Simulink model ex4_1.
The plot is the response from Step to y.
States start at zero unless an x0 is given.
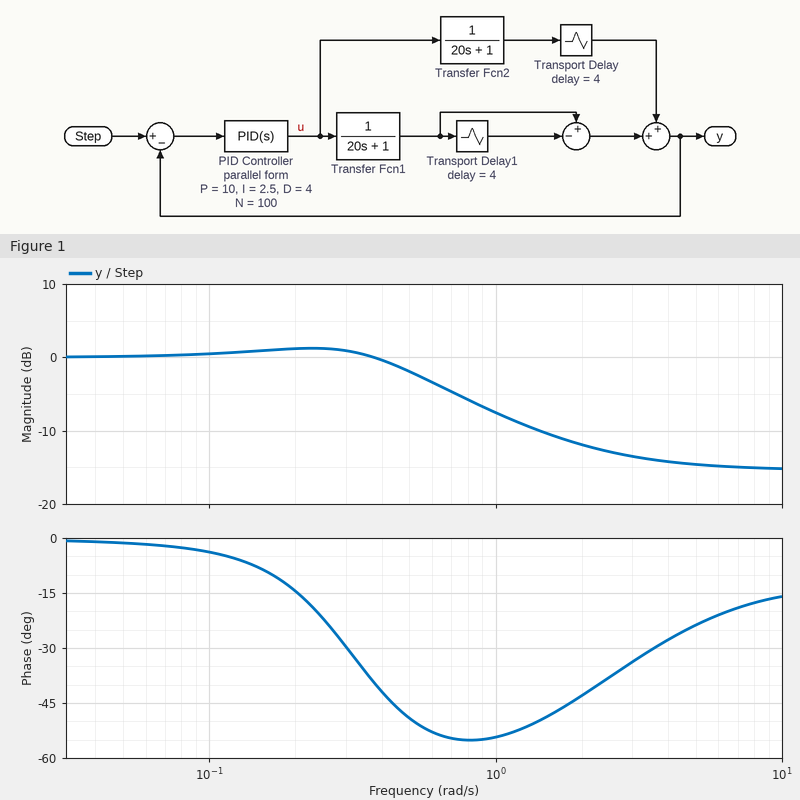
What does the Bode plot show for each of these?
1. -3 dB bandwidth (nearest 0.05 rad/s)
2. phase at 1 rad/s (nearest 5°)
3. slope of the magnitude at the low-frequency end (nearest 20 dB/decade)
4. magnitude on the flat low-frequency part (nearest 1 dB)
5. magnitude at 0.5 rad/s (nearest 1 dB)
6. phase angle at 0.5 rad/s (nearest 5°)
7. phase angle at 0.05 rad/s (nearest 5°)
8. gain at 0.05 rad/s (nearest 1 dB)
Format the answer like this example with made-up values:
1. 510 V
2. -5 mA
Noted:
1. 0.55 rad/s
2. -55°
3. 0 dB/decade
4. 0 dB
5. -2 dB
6. -50°
7. 0°
8. 0 dB
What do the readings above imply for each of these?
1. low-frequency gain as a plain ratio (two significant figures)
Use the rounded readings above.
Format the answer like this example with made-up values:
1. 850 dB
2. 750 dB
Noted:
1. 1.0
